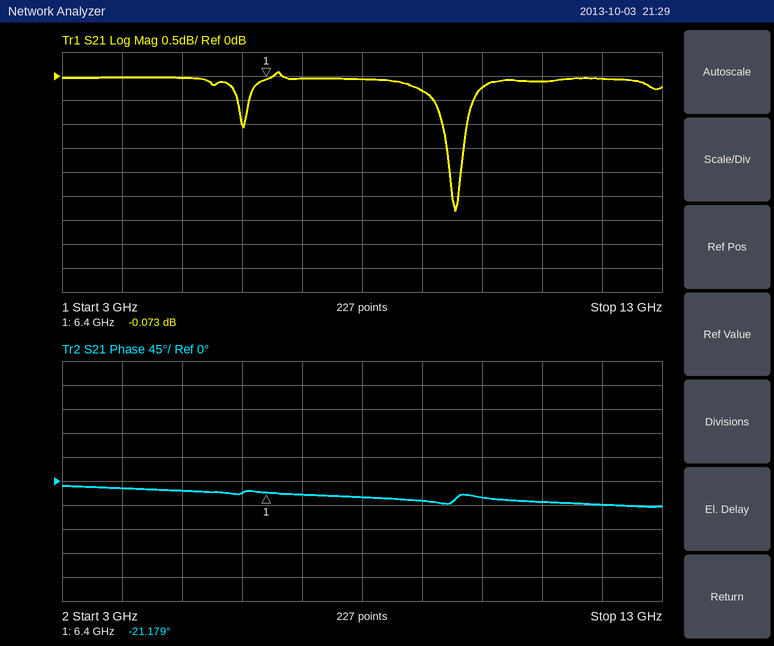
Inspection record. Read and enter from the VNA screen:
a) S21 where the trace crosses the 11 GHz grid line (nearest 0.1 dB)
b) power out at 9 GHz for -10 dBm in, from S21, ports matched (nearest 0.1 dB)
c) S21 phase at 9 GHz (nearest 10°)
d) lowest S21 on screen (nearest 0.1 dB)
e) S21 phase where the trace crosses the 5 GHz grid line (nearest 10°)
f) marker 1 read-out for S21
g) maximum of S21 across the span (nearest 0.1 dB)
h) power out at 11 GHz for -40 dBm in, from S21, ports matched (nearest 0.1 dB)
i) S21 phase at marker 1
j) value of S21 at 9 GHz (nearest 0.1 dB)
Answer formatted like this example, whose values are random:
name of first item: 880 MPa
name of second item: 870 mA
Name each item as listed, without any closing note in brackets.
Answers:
S21 where the trace crosses the 11 GHz grid line: -0.1 dB
power out at 9 GHz for -10 dBm in, from S21, ports matched: -10.3 dBm
S21 phase at 9 GHz: -40°
lowest S21 on screen: -2.8 dB
S21 phase where the trace crosses the 5 GHz grid line: -20°
marker 1 read-out for S21: -0.073 dB
maximum of S21 across the span: 0.1 dB
power out at 11 GHz for -40 dBm in, from S21, ports matched: -40.1 dBm
S21 phase at marker 1: -21.179°
value of S21 at 9 GHz: -0.3 dB
